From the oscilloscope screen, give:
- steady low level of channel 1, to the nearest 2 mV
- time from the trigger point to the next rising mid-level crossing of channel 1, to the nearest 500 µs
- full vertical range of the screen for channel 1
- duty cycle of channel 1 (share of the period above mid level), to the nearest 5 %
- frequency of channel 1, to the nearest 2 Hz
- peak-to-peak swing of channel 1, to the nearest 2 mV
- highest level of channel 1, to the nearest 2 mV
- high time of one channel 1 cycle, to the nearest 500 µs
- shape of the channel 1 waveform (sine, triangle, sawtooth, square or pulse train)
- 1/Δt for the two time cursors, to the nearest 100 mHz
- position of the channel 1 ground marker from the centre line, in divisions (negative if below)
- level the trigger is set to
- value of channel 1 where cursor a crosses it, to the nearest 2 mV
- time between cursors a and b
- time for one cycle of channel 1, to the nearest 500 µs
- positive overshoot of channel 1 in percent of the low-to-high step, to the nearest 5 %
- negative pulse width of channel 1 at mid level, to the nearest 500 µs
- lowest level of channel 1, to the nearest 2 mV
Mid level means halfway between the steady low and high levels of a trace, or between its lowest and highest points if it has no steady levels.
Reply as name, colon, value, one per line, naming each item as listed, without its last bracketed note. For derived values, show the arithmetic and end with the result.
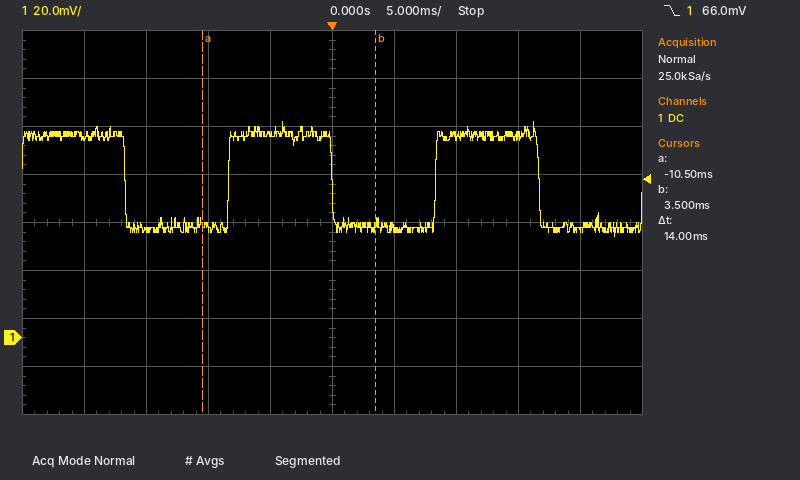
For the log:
steady low level of channel 1, to the nearest 2 mV: 46 mV
time from the trigger point to the next rising mid-level crossing of channel 1, to the nearest 500 µs: 8.5 ms
full vertical range of the screen for channel 1: 160 mV
duty cycle of channel 1 (share of the period above mid level), to the nearest 5 %: 8.5 ms / 16.5 ms ≈ 51.5 %, so 50 % to the nearest 5 %
frequency of channel 1, to the nearest 2 Hz: 1 / 16.5 ms ≈ 60.6 Hz, so 60 Hz to the nearest 2 Hz
peak-to-peak swing of channel 1, to the nearest 2 mV: 90 mV − (42 mV) = 48 mV
highest level of channel 1, to the nearest 2 mV: 90 mV
high time of one channel 1 cycle, to the nearest 500 µs: 8.5 ms
shape of the channel 1 waveform: square
1/Δt for the two time cursors, to the nearest 100 mHz: 1 / 14 ms ≈ 71.4 Hz
position of the channel 1 ground marker from the centre line, in divisions: -2.4 div
level the trigger is set to: 66.0 mV
value of channel 1 where cursor a crosses it, to the nearest 2 mV: 48 mV
time between cursors a and b: 14 ms
time for one cycle of channel 1, to the nearest 500 µs: 16.5 ms
positive overshoot of channel 1 in percent of the low-to-high step, to the nearest 5 %: 15 %
negative pulse width of channel 1 at mid level, to the nearest 500 µs: 8.5 ms
lowest level of channel 1, to the nearest 2 mV: 42 mV
